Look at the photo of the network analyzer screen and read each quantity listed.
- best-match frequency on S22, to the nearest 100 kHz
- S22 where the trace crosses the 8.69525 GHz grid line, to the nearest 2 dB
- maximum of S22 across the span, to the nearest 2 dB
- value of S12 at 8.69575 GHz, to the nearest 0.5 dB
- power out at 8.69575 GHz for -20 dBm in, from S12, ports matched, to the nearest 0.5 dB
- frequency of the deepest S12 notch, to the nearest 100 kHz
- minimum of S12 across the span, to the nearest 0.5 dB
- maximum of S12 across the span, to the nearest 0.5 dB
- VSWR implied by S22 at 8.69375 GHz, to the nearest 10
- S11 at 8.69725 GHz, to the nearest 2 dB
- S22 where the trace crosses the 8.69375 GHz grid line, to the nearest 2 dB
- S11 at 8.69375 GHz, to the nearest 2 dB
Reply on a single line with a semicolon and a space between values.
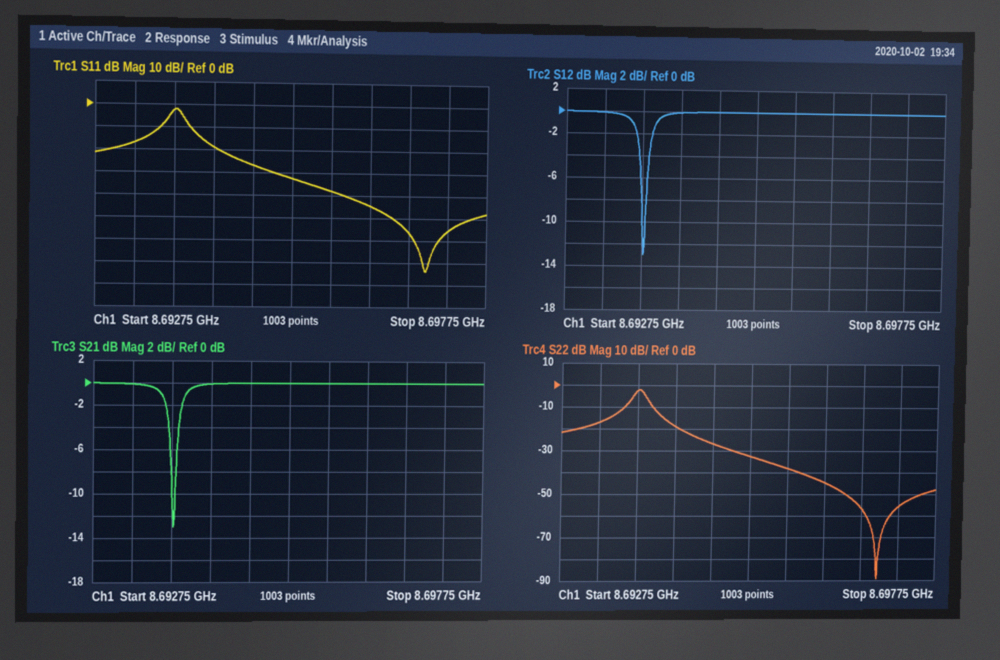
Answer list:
8.6970 GHz; -32 dB; -2 dB; 0.0 dB; -20.0 dBm; 8.6938 GHz; -13.0 dB; 0.0 dB; 10; -56 dB; -2 dB; -2 dB
